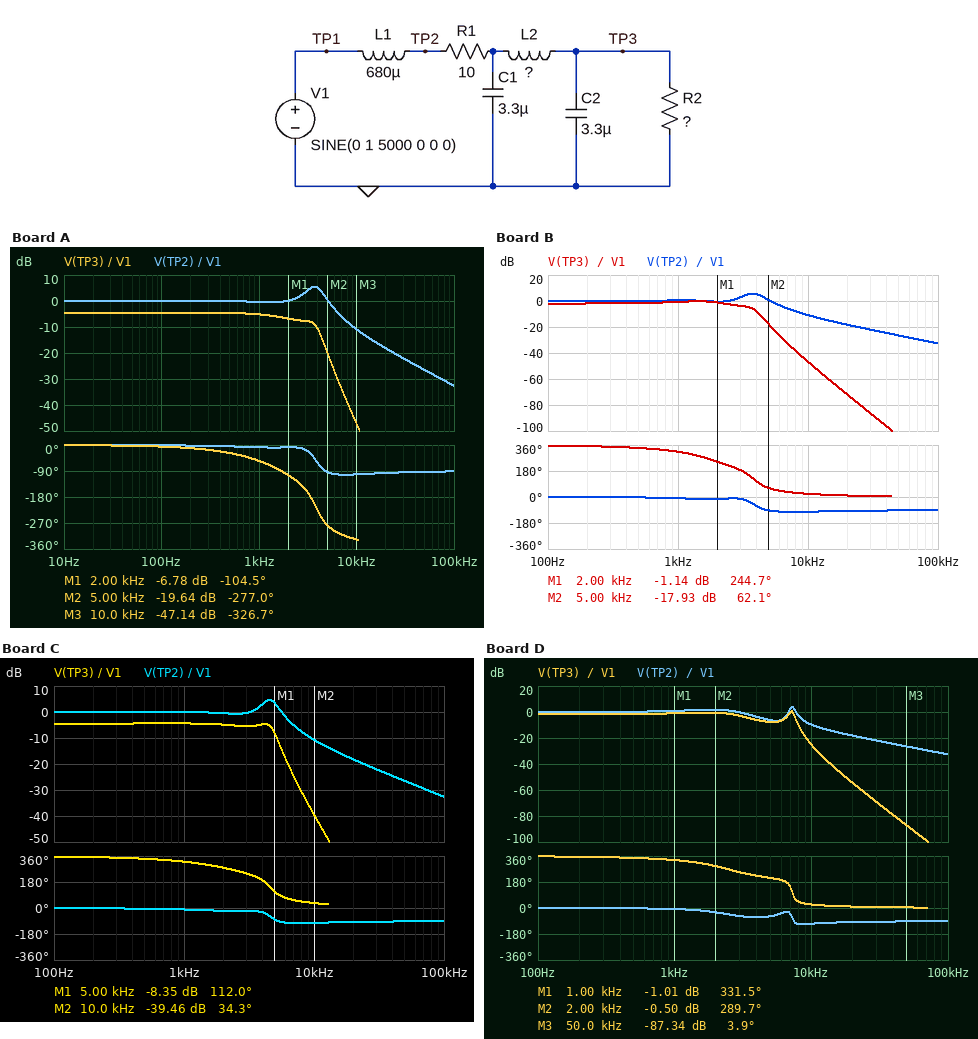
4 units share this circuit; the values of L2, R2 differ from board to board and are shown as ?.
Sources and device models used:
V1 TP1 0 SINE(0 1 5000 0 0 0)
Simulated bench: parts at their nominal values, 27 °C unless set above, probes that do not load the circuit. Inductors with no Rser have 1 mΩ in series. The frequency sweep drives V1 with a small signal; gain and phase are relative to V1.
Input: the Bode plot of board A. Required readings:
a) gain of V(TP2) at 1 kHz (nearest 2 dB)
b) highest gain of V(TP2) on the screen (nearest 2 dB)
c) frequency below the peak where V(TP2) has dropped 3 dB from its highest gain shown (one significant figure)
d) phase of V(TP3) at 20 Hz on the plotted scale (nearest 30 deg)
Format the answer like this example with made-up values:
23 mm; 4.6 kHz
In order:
0 dB; 6 dB; 3 kHz; 0 deg
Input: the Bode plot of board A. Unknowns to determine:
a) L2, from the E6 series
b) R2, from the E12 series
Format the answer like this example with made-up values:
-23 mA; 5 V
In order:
2.2 mH; 15 Ω
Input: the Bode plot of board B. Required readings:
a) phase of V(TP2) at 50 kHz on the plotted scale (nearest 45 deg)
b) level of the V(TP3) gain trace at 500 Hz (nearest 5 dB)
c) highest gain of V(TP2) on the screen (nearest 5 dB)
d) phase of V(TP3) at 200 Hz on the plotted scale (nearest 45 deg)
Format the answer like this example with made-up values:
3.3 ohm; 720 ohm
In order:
-90 deg; 0 dB; 5 dB; 360 deg
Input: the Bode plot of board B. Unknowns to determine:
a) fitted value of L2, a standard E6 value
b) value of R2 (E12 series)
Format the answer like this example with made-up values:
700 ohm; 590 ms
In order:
2.2 mH; 39 Ω
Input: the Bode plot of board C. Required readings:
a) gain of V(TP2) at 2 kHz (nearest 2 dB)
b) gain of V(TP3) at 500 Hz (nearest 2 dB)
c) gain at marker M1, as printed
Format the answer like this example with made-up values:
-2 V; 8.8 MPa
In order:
0 dB; -4 dB; -8.35 dB
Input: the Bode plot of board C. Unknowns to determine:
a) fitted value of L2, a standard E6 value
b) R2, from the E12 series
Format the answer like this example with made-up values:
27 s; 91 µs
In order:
1 mH; 15 Ω
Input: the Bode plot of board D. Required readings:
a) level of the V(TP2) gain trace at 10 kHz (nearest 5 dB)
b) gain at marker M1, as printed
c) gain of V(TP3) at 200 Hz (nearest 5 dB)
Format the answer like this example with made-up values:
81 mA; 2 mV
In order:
-10 dB; -1.01 dB; 0 dB
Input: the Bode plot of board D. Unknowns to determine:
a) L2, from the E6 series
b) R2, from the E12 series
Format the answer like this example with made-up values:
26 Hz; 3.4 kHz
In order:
330 µH; 47 Ω
